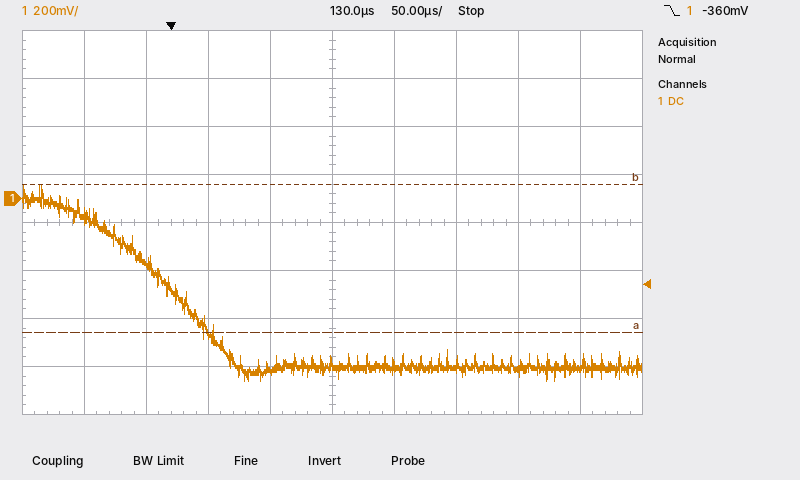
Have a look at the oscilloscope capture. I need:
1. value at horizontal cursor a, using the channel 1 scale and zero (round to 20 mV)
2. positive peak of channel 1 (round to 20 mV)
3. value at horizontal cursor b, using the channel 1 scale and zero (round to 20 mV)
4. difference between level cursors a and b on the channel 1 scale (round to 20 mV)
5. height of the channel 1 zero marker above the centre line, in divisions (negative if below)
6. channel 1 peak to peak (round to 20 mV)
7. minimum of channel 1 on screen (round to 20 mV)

-560 mV
60 mV
60 mV
620 mV
+0.5 div
820 mV
-760 mV
